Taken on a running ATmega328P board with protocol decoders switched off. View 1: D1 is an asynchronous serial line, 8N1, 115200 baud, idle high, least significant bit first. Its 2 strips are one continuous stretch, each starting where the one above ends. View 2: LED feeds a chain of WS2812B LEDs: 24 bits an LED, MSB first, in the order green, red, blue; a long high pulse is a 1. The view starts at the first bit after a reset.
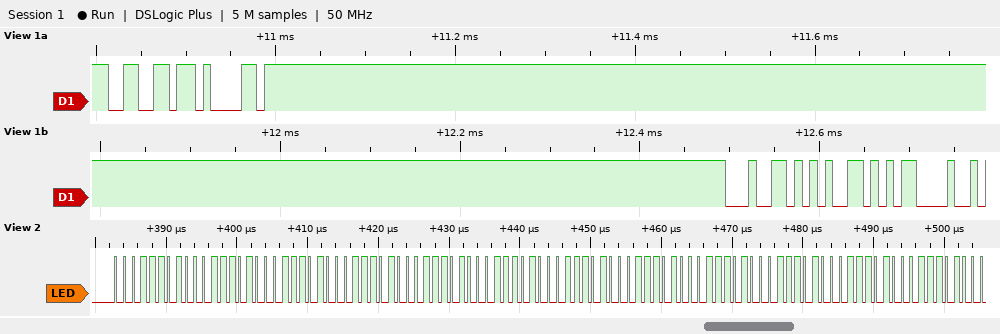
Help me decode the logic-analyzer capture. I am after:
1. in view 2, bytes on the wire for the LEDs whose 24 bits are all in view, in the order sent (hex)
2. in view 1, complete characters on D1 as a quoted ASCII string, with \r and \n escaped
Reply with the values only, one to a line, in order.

1D 1D 1D 1D 1D 1D 1D 1D 1D 1D 1D 1D
"fade\r"
